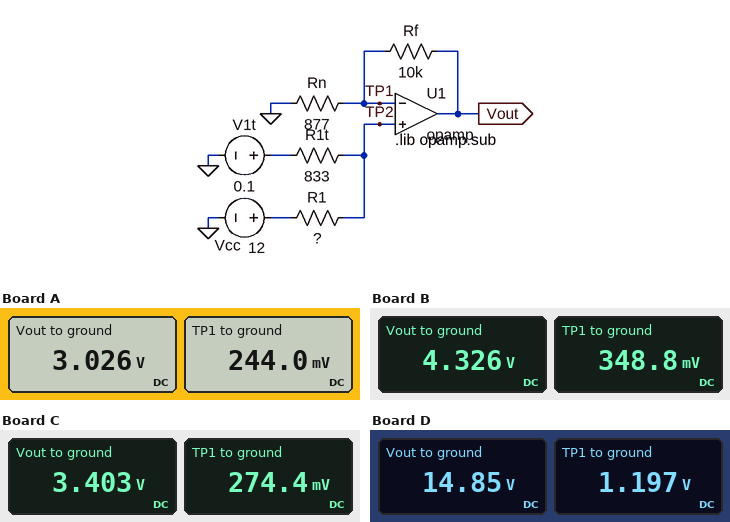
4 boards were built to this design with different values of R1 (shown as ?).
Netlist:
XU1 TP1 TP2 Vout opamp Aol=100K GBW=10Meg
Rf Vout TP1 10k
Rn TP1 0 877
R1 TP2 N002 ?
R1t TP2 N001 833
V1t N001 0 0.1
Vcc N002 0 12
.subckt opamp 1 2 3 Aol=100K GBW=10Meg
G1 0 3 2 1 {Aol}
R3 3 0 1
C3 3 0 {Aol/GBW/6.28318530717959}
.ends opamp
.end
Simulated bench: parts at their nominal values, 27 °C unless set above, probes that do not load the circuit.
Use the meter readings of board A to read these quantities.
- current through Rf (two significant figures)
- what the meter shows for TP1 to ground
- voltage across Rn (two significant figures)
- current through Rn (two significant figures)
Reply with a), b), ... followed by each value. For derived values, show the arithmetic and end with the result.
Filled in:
a) (3.026 V - 244 mV) / 10 kΩ = 280 µA
b) 244.0 mV
c) 244 mV = 240 mV
d) (244 mV) / 877 Ω = 280 µA
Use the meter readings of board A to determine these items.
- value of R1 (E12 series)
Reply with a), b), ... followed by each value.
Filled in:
a) 68 kΩ
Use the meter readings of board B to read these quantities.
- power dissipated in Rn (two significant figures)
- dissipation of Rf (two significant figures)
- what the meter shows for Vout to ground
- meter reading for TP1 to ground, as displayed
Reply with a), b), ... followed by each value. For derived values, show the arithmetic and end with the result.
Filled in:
a) (348.8 mV)^2 / 877 Ω = 140 µW
b) (4.326 V - 348.8 mV)^2 / 10 kΩ = 1.6 mW
c) 4.326 V
d) 348.8 mV
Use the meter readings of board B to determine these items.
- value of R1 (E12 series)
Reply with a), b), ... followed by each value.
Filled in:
a) 39 kΩ
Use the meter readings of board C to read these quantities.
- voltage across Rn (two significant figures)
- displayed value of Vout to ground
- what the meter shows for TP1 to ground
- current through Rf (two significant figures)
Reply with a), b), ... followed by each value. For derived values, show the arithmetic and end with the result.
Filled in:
a) 274.4 mV = 270 mV
b) 3.403 V
c) 274.4 mV
d) (3.403 V - 274.4 mV) / 10 kΩ = 310 µA
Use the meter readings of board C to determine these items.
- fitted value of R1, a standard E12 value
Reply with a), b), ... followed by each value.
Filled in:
a) 56 kΩ
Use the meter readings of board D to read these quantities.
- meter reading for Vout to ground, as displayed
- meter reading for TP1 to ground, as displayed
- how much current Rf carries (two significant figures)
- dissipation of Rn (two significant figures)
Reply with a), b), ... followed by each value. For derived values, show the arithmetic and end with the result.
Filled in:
a) 14.85 V
b) 1.197 V
c) (14.85 V - 1.197 V) / 10 kΩ = 1.4 mA
d) (1.197 V)^2 / 877 Ω = 1.6 mW
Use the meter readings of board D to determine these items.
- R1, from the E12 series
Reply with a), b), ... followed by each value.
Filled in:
a) 8.2 kΩ
